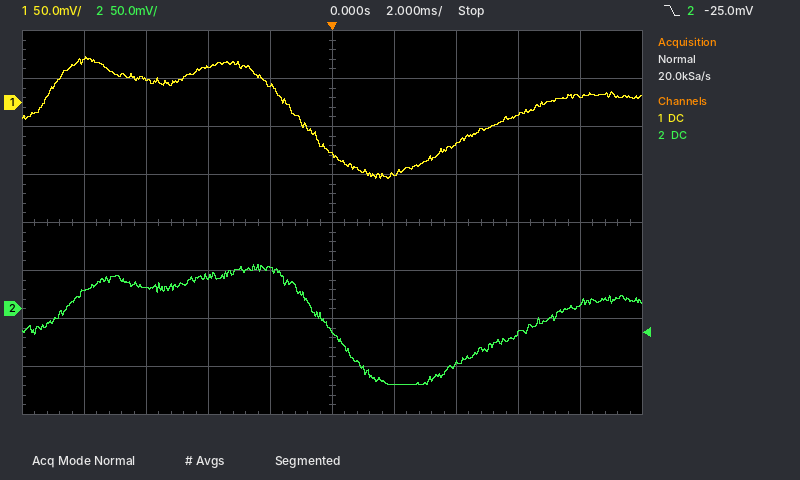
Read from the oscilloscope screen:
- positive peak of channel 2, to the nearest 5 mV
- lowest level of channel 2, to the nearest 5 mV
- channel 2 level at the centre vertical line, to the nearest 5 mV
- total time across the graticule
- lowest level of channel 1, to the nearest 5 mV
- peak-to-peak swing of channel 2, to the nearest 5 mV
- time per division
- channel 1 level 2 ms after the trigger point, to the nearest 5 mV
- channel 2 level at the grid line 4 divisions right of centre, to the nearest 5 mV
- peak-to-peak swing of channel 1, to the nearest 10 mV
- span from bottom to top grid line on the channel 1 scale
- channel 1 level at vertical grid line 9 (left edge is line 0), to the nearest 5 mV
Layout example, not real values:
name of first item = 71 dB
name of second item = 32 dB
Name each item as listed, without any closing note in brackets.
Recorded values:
positive peak of channel 2, to the nearest 5 mV = 45 mV
lowest level of channel 2, to the nearest 5 mV = -80 mV
channel 2 level at the centre vertical line, to the nearest 5 mV = -25 mV
total time across the graticule = 20 ms
lowest level of channel 1, to the nearest 5 mV = -80 mV
peak-to-peak swing of channel 2, to the nearest 5 mV = 125 mV
time per division = 2 ms
channel 1 level 2 ms after the trigger point, to the nearest 5 mV = -75 mV
channel 2 level at the grid line 4 divisions right of centre, to the nearest 5 mV = 5 mV
peak-to-peak swing of channel 1, to the nearest 10 mV = 130 mV
span from bottom to top grid line on the channel 1 scale = 400 mV
channel 1 level at vertical grid line 9 (left edge is line 0), to the nearest 5 mV = 5 mV
